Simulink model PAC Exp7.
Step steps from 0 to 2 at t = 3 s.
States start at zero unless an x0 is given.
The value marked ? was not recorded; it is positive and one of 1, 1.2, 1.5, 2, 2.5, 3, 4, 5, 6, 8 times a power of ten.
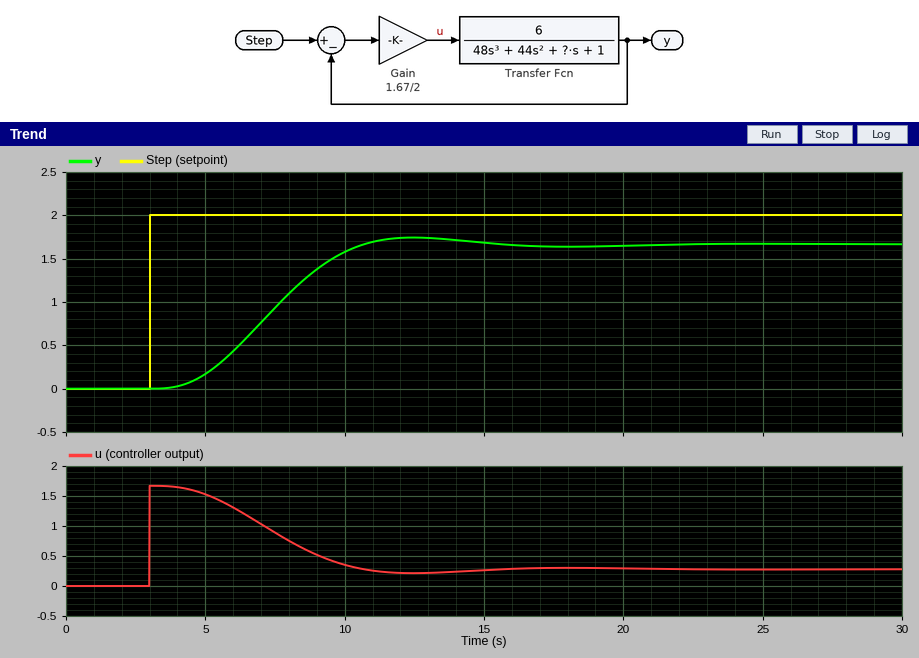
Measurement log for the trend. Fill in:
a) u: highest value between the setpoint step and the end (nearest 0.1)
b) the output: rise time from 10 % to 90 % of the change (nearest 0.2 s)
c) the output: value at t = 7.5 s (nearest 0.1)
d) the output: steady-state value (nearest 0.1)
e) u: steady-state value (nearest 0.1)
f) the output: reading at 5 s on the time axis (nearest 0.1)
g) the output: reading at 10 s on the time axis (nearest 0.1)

1.7
4.6 s
0.9
1.7
0.3
0.2
1.6
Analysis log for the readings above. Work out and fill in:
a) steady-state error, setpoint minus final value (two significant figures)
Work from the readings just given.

0.30
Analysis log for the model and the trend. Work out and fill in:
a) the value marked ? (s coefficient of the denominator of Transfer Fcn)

25
